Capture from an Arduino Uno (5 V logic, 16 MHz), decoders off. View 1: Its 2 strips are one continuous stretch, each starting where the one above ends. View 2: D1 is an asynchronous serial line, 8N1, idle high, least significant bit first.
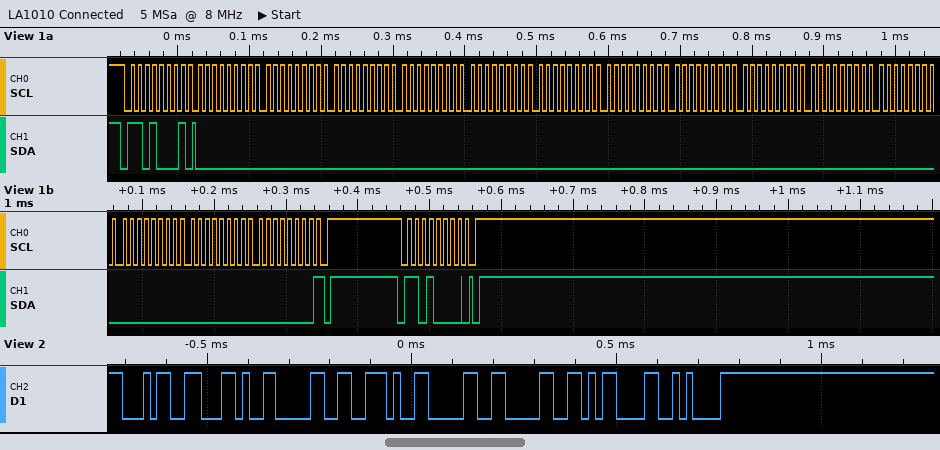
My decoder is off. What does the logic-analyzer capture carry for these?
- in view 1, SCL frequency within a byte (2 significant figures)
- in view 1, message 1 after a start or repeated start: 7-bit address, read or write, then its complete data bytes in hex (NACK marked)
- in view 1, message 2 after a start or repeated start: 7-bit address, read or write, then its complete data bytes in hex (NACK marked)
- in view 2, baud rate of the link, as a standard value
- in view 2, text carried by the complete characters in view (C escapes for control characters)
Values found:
100 kHz
0x68 read: 00 00 00 00 00 00 00 00 00 00 00 00 00 00 NACK
0x68 write
57600 baud
"4,0.00\r\n"
